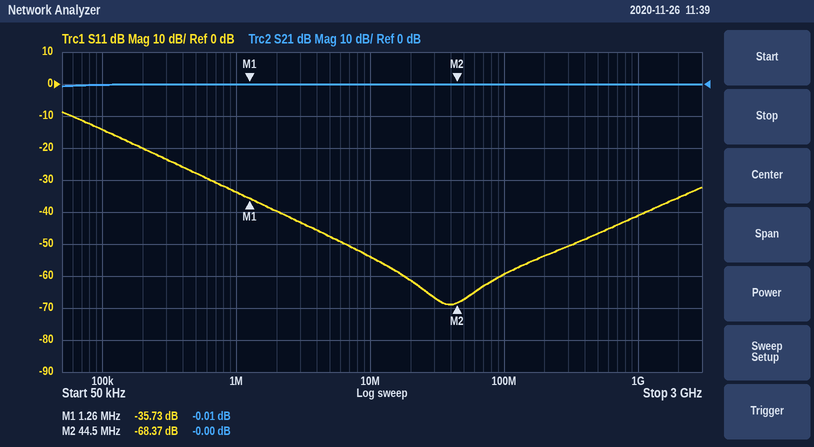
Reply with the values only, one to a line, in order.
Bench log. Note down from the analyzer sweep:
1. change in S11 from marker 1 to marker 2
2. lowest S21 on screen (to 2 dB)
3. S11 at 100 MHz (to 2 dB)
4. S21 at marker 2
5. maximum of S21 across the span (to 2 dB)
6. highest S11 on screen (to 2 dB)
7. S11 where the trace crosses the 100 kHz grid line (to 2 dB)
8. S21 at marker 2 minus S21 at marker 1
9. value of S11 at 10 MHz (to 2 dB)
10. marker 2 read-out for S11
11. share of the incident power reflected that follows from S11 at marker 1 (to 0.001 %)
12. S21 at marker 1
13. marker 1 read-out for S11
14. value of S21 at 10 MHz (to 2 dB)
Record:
-32.64 dB
0 dB
-60 dB
-0.00 dB
0 dB
-8 dB
-14 dB
0.01 dB
-54 dB
-68.37 dB
0.027 %
-0.01 dB
-35.73 dB
0 dB
